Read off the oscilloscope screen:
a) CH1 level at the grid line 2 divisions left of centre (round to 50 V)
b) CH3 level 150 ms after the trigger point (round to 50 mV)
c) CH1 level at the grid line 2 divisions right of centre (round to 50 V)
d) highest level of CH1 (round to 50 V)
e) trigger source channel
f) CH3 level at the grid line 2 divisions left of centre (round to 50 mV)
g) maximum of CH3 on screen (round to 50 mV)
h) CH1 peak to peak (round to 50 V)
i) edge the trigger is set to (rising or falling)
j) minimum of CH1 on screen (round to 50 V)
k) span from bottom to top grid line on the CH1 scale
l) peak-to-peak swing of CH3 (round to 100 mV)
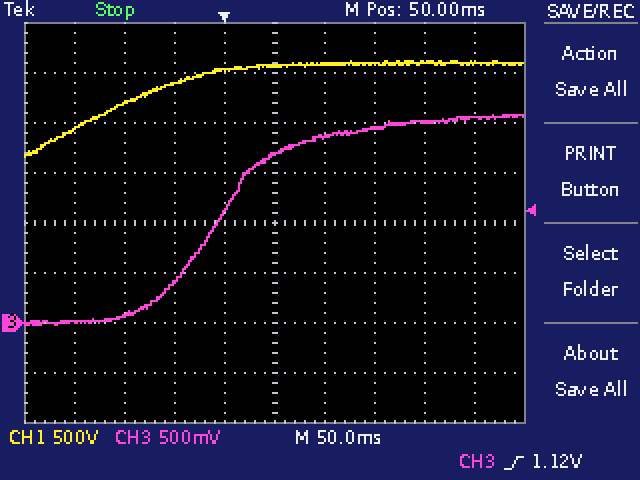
2.40 kV
1.95 V
2.60 kV
2.60 kV
CH3
400 mV
2.10 V
950 V
rising
1.65 kV
4 kV
2.10 V
